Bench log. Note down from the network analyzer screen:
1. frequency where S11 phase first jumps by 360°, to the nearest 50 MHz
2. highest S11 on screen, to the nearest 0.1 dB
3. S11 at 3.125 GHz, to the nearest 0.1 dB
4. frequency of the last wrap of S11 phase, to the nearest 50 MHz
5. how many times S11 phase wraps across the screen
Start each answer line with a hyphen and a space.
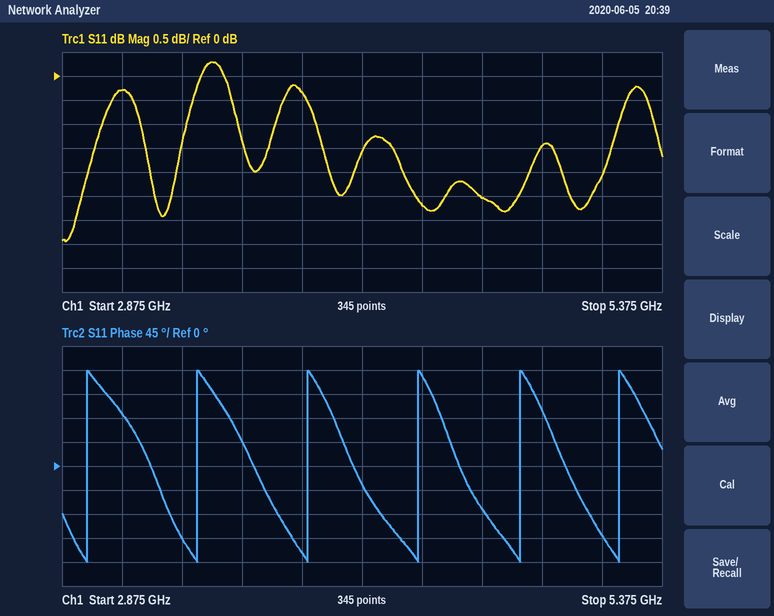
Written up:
- 3.00 GHz
- 0.3 dB
- -0.3 dB
- 5.20 GHz
- 6
